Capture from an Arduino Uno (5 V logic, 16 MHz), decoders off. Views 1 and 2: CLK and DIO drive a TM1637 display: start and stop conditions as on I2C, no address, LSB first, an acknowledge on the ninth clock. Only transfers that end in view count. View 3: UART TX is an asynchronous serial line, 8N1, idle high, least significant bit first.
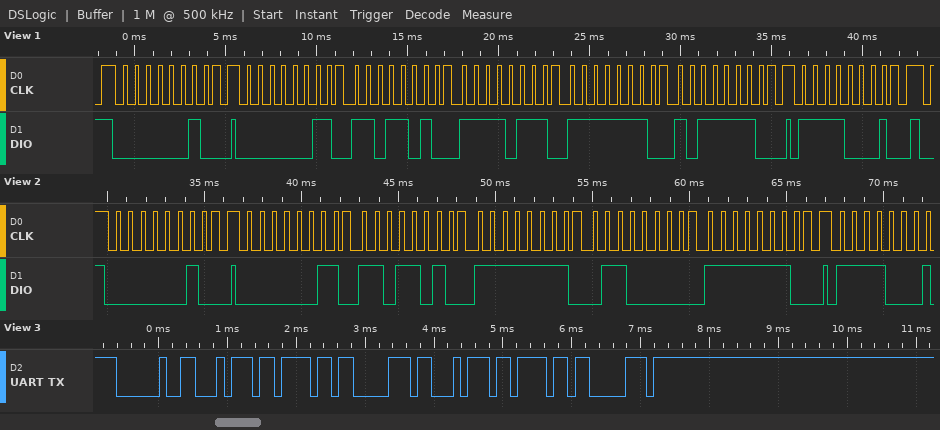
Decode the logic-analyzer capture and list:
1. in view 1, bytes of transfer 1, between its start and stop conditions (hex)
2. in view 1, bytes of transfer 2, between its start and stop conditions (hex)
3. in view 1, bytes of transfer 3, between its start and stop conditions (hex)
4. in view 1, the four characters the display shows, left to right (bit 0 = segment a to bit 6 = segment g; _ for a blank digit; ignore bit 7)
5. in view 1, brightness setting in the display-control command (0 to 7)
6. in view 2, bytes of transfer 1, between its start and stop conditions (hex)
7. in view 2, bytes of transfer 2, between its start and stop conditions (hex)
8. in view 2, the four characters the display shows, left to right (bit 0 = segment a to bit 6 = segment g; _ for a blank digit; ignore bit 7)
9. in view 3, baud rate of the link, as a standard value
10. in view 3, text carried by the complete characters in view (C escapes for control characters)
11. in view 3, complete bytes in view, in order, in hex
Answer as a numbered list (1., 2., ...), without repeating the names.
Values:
1. 40
2. C0 5B EF 7F 7D
3. 8F
4. 2986
5. 7
6. 40
7. C0 5B FF 06 7F
8. 2818
9. 9600 baud
10. " toptop"
11. 20 74 6F 70 74 6F 70
